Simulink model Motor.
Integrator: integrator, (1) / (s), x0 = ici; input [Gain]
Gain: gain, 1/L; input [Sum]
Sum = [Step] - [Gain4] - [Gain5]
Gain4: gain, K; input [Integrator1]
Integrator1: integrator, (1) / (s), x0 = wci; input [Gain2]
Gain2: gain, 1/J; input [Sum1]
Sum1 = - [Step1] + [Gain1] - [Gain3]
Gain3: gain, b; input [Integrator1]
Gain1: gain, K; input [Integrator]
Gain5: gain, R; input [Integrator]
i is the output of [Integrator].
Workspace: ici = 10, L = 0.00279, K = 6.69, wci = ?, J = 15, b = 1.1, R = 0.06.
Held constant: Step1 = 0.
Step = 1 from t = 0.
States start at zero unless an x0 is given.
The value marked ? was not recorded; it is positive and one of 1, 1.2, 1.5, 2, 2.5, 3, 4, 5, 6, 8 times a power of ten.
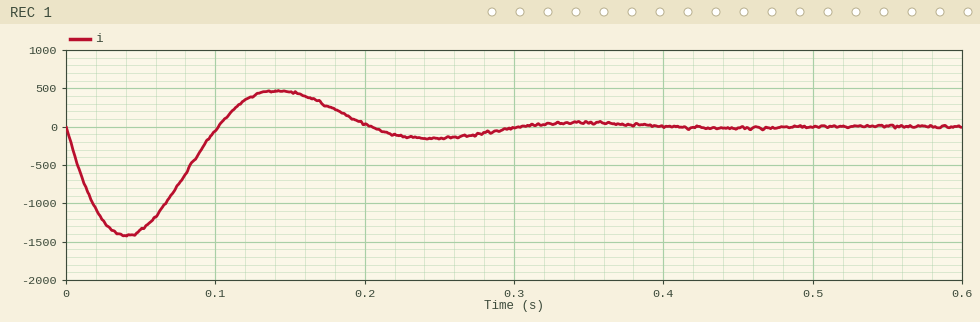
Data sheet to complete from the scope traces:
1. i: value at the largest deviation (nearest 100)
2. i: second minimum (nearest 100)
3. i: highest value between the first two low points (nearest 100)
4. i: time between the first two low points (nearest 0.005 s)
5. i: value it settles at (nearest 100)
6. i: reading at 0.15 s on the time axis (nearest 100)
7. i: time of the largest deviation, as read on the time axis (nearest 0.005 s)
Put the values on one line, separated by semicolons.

-1400; -200; 500; 0.205 s; 0; 500; 0.040 s
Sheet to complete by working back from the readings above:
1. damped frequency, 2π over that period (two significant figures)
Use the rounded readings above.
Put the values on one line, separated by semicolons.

31 rad/s
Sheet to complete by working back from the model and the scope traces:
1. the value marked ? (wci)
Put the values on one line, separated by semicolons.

30
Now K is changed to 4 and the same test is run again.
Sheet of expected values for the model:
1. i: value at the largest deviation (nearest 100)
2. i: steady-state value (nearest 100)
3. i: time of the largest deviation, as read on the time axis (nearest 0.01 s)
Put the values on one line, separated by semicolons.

-1100; 0; 0.06 s
